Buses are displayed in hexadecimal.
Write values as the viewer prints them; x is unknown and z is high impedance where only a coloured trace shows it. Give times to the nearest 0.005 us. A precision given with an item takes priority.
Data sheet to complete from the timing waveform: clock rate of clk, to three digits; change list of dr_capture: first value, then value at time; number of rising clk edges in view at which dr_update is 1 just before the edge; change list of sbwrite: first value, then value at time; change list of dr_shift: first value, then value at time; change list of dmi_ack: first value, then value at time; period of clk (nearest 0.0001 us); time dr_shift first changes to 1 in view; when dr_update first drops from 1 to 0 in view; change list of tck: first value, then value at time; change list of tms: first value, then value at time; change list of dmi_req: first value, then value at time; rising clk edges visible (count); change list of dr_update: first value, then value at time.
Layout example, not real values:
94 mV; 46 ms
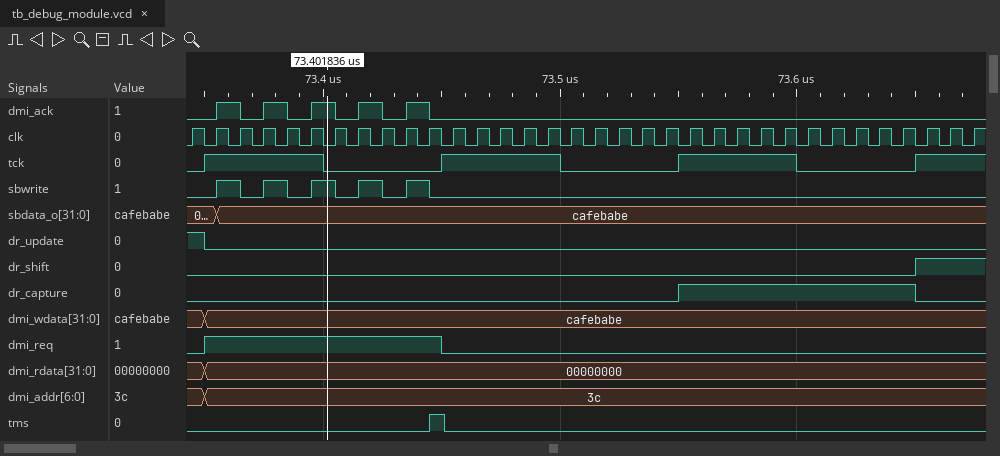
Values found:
100 MHz; 0, 1 at 73.55 us, 0 at 73.65 us; 1; 0, 1 at 73.355 us, 0 at 73.365 us, 1 at 73.375 us, 0 at 73.385 us, 1 at 73.395 us, 0 at 73.405 us, 1 at 73.415 us, 0 at 73.425 us, 1 at 73.435 us, 0 at 73.445 us; 0, 1 at 73.65 us; 0, 1 at 73.355 us, 0 at 73.365 us, 1 at 73.375 us, 0 at 73.385 us, 1 at 73.395 us, 0 at 73.405 us, 1 at 73.415 us, 0 at 73.425 us, 1 at 73.435 us, 0 at 73.445 us; 0.01 us; 73.65 us; 73.35 us; 0, 1 at 73.35 us, 0 at 73.4 us, 1 at 73.45 us, 0 at 73.5 us, 1 at 73.55 us, 0 at 73.6 us, 1 at 73.65 us; 0, 1 at 73.445 us, 0 at 73.45 us; 0, 1 at 73.35 us, 0 at 73.45 us; 34; 1, 0 at 73.35 us
